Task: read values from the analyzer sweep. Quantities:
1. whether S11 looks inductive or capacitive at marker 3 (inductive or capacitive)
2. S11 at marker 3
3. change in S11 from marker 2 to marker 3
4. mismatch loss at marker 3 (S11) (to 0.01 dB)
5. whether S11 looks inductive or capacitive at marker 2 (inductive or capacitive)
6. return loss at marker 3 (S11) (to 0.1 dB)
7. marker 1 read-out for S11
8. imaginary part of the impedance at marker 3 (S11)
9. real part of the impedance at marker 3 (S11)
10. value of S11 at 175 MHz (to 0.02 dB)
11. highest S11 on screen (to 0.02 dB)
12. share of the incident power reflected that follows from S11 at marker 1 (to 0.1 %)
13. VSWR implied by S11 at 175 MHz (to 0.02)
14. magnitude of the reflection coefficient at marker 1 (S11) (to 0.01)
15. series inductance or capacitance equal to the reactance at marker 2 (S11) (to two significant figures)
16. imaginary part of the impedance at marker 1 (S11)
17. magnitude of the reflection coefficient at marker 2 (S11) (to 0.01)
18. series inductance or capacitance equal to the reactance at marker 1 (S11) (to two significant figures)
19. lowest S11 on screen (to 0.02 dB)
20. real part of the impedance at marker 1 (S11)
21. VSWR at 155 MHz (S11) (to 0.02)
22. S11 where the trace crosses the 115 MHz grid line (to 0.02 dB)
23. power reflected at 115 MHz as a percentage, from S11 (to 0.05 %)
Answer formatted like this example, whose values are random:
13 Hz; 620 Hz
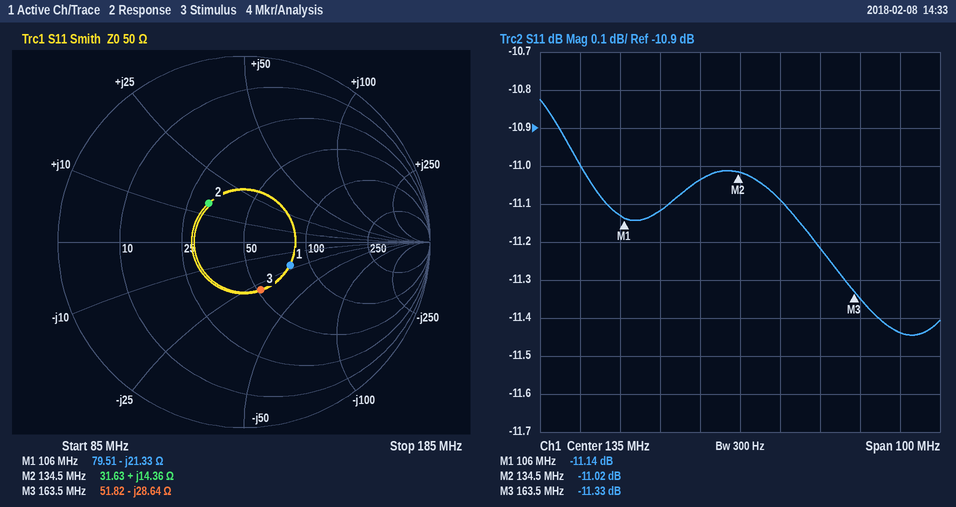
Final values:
capacitive; -11.33 dB; -0.31 dB; 0.33 dB; inductive; 11.3 dB; -11.14 dB; -28.64 Ω; 51.82 Ω; -11.44 dB; -10.82 dB; 7.7 %; 1.74; 0.28; 17 nH; -21.33 Ω; 0.28; 70 pF; -11.44 dB; 79.51 Ω; 1.76; -11.12 dB; 7.75 %
